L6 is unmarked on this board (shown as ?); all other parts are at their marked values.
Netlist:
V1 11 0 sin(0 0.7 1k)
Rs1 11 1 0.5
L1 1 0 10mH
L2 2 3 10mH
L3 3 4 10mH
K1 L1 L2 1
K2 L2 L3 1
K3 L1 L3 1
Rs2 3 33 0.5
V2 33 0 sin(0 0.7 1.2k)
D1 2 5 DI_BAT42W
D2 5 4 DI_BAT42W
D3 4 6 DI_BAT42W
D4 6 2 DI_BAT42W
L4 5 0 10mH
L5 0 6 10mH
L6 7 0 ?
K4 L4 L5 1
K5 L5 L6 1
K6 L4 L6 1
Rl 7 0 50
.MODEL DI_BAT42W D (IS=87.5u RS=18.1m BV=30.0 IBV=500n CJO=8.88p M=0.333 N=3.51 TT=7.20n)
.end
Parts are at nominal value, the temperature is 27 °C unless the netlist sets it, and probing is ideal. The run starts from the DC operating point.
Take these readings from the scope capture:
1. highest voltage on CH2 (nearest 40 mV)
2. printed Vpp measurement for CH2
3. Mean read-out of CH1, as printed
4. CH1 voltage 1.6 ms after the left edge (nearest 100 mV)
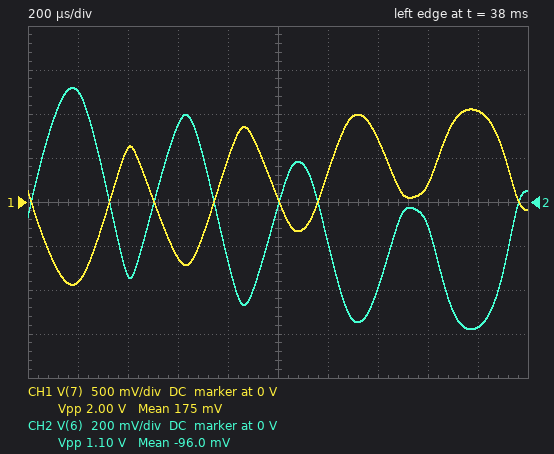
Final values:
520 mV
1.10 V
175 mV
200 mV
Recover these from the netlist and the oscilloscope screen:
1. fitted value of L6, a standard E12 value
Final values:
33 mH
